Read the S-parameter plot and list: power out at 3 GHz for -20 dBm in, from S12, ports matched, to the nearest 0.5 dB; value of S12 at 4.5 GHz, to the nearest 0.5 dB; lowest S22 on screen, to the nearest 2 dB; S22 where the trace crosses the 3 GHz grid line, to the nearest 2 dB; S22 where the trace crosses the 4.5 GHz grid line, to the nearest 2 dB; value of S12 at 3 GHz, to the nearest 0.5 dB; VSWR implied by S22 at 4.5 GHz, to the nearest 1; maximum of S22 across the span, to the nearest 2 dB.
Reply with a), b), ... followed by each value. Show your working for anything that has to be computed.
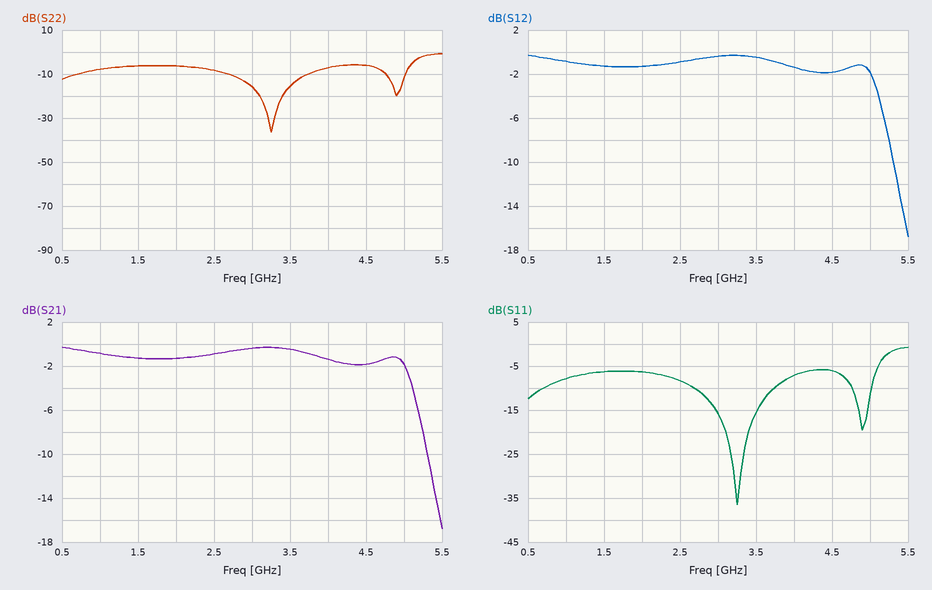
a) -20 dBm + (-0.5 dB) = -20.5 dBm
b) -2.0 dB
c) -36 dB
d) -16 dB
e) -6 dB
f) -0.5 dB
g) |Γ| = 10^(-6/20) = 0.5012; VSWR = (1 + 0.5012)/(1 − 0.5012) ≈ 3
h) 0 dB
